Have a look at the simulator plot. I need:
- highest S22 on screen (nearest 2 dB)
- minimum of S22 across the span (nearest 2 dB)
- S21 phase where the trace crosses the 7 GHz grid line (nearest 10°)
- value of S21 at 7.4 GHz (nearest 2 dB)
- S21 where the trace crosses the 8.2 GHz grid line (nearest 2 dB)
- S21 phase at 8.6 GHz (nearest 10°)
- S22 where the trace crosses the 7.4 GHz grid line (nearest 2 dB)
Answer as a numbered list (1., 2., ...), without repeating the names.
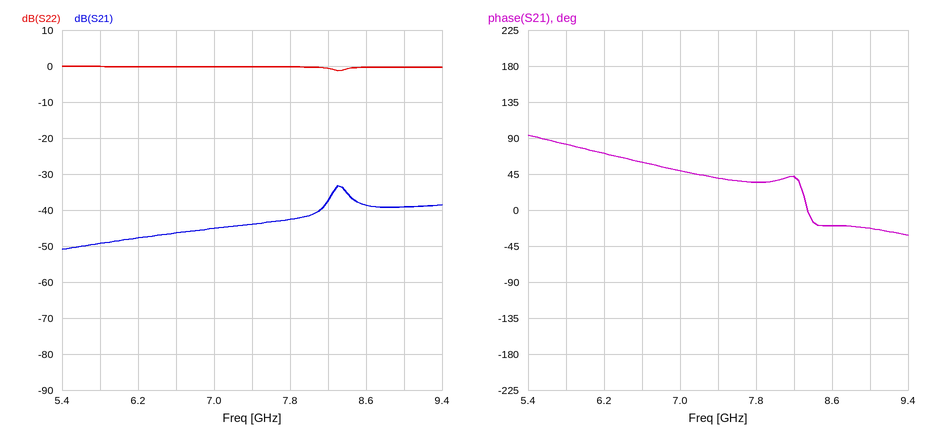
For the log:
1. 0 dB
2. -2 dB
3. 50°
4. -44 dB
5. -38 dB
6. -20°
7. 0 dB
